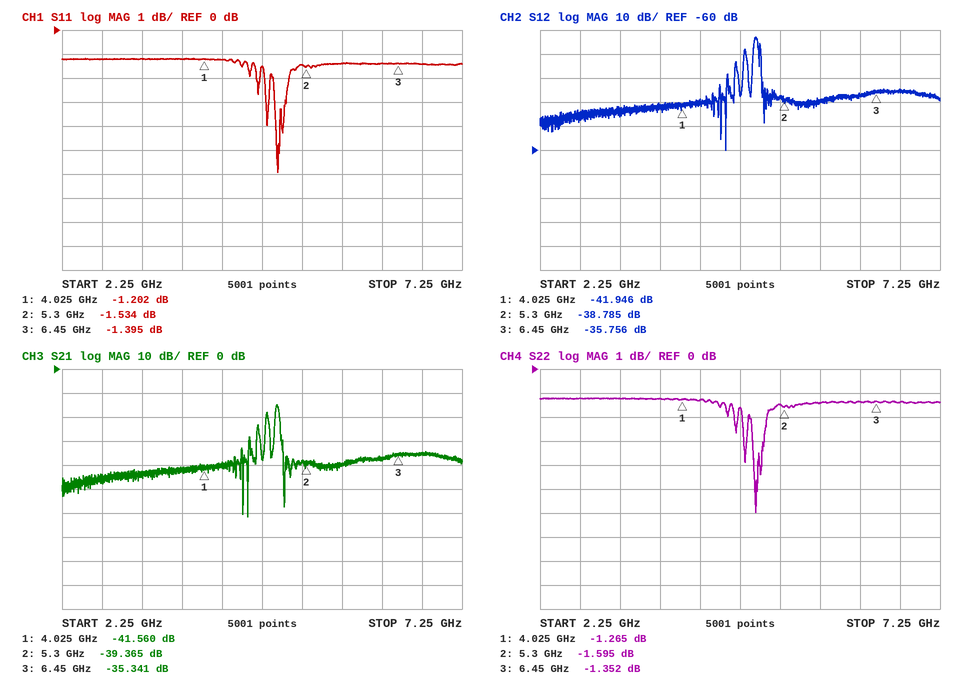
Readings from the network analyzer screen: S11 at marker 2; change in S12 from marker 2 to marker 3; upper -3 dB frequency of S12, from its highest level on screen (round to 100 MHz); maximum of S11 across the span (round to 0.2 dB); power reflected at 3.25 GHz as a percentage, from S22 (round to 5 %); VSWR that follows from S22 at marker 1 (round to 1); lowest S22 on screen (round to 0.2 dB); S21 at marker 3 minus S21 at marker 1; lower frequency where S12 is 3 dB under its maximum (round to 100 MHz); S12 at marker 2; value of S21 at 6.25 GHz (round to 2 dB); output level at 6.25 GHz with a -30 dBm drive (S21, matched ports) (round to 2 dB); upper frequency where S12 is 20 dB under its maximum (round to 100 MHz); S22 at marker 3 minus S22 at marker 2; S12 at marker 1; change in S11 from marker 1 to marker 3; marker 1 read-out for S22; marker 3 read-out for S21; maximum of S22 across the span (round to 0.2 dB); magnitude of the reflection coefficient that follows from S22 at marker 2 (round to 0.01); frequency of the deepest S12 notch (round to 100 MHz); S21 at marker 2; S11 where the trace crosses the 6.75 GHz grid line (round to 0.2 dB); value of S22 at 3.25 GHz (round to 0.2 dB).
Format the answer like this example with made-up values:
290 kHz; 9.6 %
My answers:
-1.534 dB; 3.029 dB; 5.0 GHz; -1.2 dB; 75 %; 14; -6.0 dB; 6.219 dB; 4.9 GHz; -38.785 dB; -38 dB; -68 dBm; 5.0 GHz; 0.243 dB; -41.946 dB; -0.193 dB; -1.265 dB; -35.341 dB; -1.2 dB; 0.83; 4.6 GHz; -39.365 dB; -1.4 dB; -1.2 dB
